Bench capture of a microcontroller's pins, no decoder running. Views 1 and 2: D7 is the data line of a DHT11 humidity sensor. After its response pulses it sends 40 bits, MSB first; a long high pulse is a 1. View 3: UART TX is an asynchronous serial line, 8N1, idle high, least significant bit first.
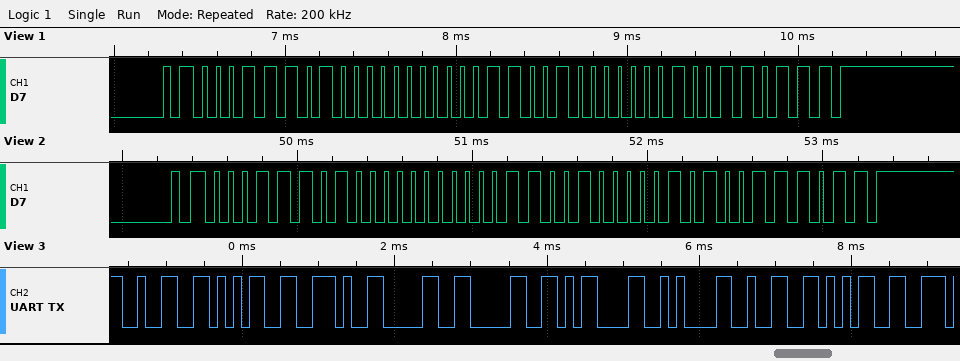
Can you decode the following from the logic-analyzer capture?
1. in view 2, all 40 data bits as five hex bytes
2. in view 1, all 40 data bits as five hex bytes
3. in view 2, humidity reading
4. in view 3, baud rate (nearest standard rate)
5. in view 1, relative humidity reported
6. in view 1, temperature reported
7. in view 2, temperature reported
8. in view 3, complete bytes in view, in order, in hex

1D 00 19 05 3B
1D 00 19 01 37
29 %
9600 baud
29 %
25.1 °C
25.5 °C
32 35 2E 30 30 0D 0A 32 35
